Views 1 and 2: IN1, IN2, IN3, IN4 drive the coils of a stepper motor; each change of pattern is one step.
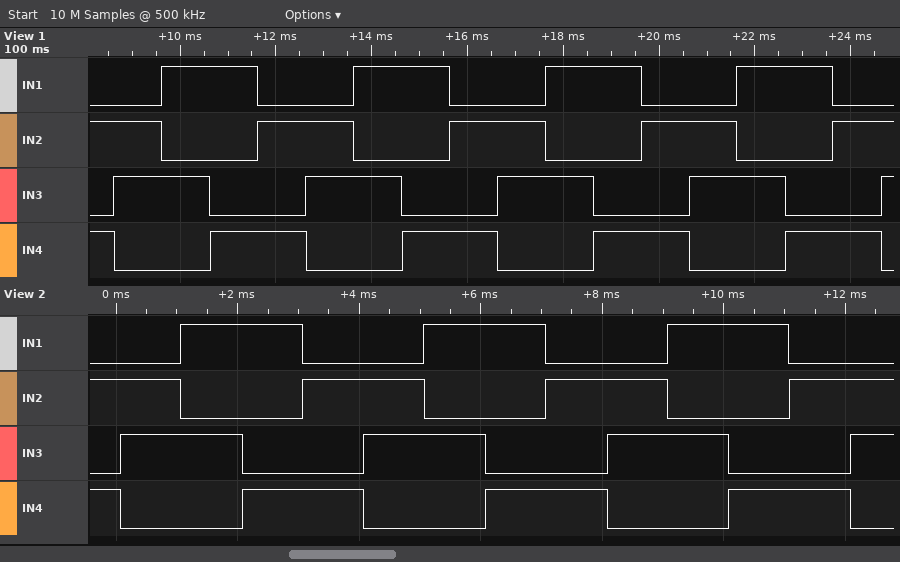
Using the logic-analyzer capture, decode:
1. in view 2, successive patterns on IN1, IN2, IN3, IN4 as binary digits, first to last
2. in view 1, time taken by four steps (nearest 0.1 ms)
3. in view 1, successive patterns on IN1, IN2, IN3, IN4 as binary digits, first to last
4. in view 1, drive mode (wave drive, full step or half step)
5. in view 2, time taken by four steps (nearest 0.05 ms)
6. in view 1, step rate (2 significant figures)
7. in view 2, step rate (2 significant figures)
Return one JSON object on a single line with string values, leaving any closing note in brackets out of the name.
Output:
{"in view 2, successive patterns on IN1, IN2, IN3, IN4 as binary digits, first to last": "0101 0110 1010 1001 0101 0110 1010 1001 0101 0110 1010 1001 0101 0110", "in view 1, time taken by four steps": "4.0 ms", "in view 1, successive patterns on IN1, IN2, IN3, IN4 as binary digits, first to last": "0101 0110 1010 1001 0101 0110 1010 1001 0101 0110 1010 1001 0101 0110 1010 1001 0101 0110", "in view 1, drive mode": "full step", "in view 2, time taken by four steps": "4.00 ms", "in view 1, step rate": "1000 steps/s", "in view 2, step rate": "1000 steps/s"}
